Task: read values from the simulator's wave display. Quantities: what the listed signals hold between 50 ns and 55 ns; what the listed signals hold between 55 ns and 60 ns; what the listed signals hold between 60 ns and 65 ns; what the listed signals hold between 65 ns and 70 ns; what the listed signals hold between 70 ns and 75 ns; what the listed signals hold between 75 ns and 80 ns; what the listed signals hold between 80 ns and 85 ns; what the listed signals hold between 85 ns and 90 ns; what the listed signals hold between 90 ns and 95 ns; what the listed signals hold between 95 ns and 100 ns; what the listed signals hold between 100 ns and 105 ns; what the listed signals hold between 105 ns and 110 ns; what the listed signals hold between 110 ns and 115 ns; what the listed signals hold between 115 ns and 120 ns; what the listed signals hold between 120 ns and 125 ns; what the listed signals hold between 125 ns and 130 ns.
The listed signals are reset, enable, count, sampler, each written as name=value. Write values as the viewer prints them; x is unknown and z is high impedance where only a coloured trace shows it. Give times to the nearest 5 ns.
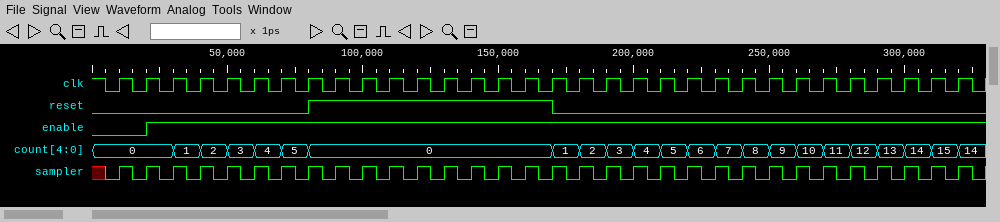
reset=0, enable=1, count=3, sampler=1
reset=0, enable=1, count=3, sampler=0
reset=0, enable=1, count=4, sampler=1
reset=0, enable=1, count=4, sampler=0
reset=0, enable=1, count=5, sampler=1
reset=0, enable=1, count=5, sampler=0
reset=1, enable=1, count=0, sampler=1
reset=1, enable=1, count=0, sampler=0
reset=1, enable=1, count=0, sampler=1
reset=1, enable=1, count=0, sampler=0
reset=1, enable=1, count=0, sampler=1
reset=1, enable=1, count=0, sampler=0
reset=1, enable=1, count=0, sampler=1
reset=1, enable=1, count=0, sampler=0
reset=1, enable=1, count=0, sampler=1
reset=1, enable=1, count=0, sampler=0
